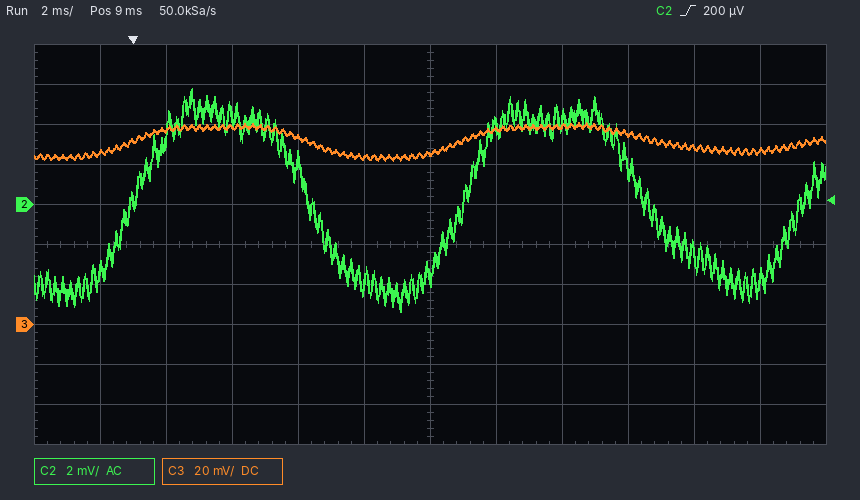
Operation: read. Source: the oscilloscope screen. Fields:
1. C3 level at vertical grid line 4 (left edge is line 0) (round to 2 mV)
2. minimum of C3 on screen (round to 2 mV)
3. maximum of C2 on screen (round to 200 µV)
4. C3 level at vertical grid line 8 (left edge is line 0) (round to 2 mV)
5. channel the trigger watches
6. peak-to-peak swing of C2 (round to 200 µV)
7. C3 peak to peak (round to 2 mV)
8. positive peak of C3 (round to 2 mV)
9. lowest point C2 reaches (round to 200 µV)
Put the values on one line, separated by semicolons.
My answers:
94 mV; 82 mV; 5.8 mV; 100 mV; C2; 11.2 mV; 18 mV; 100 mV; -5.4 mV
